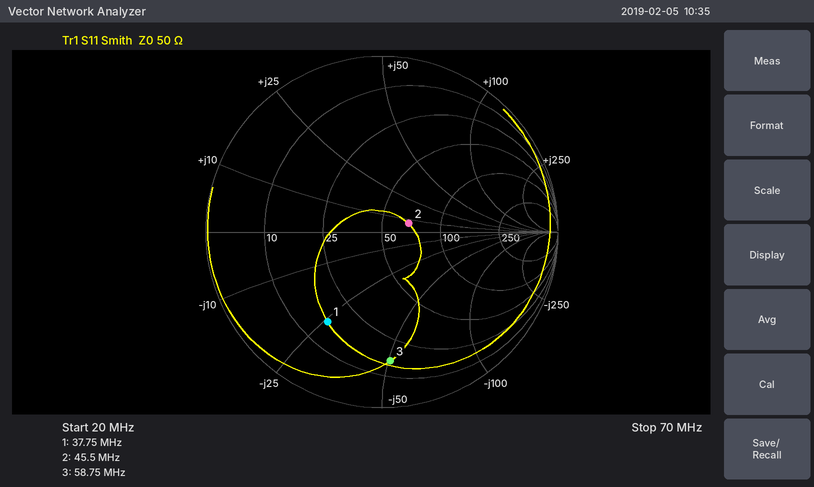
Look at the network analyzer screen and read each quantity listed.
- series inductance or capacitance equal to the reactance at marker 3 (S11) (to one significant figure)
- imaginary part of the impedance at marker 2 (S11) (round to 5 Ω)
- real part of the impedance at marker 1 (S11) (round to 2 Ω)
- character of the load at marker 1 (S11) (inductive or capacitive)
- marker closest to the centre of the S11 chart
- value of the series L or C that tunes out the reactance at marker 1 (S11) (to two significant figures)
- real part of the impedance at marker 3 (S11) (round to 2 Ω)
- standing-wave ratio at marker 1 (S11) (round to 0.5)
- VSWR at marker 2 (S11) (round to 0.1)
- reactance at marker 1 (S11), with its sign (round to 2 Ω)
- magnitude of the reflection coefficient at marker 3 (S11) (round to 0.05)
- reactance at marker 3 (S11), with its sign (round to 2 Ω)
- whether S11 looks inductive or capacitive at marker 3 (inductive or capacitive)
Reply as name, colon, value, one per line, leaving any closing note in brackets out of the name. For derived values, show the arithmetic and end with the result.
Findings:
series inductance or capacitance equal to the reactance at marker 3 (S11): C = 1/(2π × 58.75 MHz × 50 Ω) ≈ 54.2 pF, so 50 pF to one significant figure
imaginary part of the impedance at marker 2 (S11): +5 Ω
real part of the impedance at marker 1 (S11): 16 Ω
character of the load at marker 1 (S11): capacitive
marker closest to the centre of the S11 chart: marker 2
value of the series L or C that tunes out the reactance at marker 1 (S11): L = 26 Ω/(2π × 37.75 MHz) ≈ 110 nH
real part of the impedance at marker 3 (S11): 16 Ω
standing-wave ratio at marker 1 (S11): 4.0
VSWR at marker 2 (S11): 1.4
reactance at marker 1 (S11), with its sign: -26 Ω
magnitude of the reflection coefficient at marker 3 (S11): 0.75
reactance at marker 3 (S11), with its sign: -50 Ω
whether S11 looks inductive or capacitive at marker 3: capacitive
